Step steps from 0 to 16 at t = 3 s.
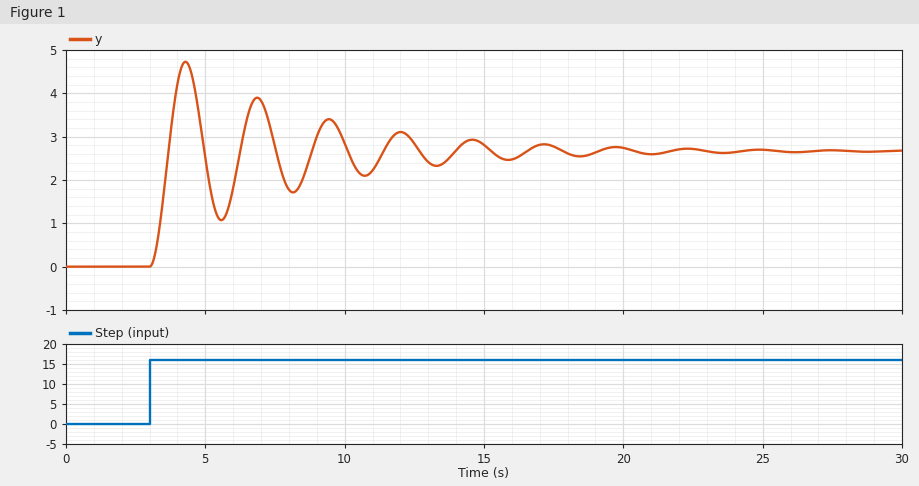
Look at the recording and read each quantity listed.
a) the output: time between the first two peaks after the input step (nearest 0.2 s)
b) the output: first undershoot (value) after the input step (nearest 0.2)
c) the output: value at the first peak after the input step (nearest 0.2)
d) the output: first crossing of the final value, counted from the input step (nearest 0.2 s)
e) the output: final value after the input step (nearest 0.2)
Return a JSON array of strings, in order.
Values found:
["2.6 s", "1.0", "4.8", "0.6 s", "2.6"]
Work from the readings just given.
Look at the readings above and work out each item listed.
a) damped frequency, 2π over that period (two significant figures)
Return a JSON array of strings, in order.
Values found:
["2.4 rad/s"]
